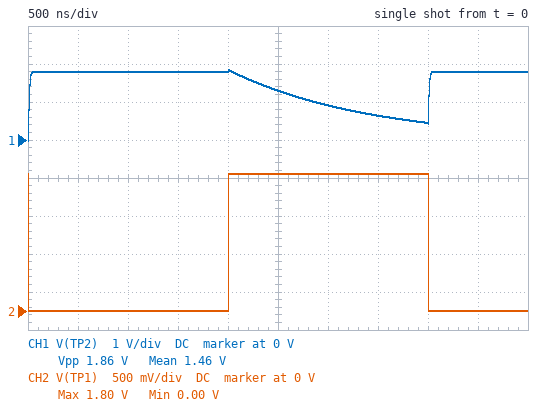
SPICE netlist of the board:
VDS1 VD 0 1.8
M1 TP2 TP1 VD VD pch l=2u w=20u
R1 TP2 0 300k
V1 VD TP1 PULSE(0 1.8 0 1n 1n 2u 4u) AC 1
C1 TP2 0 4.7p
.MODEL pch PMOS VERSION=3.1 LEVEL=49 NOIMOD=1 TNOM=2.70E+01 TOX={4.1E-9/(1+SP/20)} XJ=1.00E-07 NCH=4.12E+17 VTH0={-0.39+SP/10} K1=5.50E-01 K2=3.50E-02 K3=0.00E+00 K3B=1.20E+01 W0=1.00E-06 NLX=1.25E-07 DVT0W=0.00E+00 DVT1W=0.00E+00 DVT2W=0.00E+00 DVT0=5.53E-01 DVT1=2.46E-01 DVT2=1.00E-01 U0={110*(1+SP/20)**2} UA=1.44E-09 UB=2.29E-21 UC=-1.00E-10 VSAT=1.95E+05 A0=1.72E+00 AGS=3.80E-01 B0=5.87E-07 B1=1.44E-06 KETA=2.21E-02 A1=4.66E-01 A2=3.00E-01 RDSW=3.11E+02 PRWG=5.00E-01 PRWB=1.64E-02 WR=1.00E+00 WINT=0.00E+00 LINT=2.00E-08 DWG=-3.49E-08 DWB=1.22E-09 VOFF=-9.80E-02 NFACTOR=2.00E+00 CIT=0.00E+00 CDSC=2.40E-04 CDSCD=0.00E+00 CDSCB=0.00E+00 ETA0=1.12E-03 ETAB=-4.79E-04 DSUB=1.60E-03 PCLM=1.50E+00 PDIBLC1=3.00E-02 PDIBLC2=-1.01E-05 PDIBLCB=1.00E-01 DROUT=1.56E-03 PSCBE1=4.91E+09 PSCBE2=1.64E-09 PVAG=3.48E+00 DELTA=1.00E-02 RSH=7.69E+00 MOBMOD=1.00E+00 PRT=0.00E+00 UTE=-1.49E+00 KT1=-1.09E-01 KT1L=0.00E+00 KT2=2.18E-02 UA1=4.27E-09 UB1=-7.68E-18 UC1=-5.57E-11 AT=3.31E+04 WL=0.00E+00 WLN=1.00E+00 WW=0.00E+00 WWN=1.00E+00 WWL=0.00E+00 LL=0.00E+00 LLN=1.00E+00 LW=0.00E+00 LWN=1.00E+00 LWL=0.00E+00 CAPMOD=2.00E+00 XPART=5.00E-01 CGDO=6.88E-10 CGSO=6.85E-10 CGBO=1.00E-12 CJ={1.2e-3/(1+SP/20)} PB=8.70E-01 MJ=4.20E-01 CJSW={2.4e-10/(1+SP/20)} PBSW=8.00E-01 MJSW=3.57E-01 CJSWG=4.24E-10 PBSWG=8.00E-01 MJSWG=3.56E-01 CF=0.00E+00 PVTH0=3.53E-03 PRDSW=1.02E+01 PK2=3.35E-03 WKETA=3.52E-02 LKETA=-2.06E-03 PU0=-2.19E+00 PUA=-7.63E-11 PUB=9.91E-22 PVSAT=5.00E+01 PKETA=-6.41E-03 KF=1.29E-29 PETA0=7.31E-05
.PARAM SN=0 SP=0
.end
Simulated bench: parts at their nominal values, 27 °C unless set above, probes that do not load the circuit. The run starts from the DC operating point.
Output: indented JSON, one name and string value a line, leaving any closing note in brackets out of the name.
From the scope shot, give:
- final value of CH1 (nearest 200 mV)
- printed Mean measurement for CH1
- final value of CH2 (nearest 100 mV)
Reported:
{
  "final value of CH1": "1.8 V",
  "printed Mean measurement for CH1": "1.46 V",
  "final value of CH2": "0 V"
}
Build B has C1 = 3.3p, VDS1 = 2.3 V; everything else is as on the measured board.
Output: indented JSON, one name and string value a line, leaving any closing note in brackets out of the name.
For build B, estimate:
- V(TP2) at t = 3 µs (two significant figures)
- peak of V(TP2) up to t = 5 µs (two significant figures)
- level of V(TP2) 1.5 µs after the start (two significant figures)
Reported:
{
  "V(TP2) at t = 3 µs": "870 mV",
  "peak of V(TP2) up to t = 5 µs": "2.4 V",
  "level of V(TP2) 1.5 µs after the start": "2.3 V"
}
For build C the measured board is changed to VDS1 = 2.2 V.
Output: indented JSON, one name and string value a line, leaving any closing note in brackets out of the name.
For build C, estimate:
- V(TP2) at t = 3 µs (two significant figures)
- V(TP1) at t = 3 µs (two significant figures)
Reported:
{
  "V(TP2) at t = 3 µs": "1.1 V",
  "V(TP1) at t = 3 µs": "2.2 V"
}
